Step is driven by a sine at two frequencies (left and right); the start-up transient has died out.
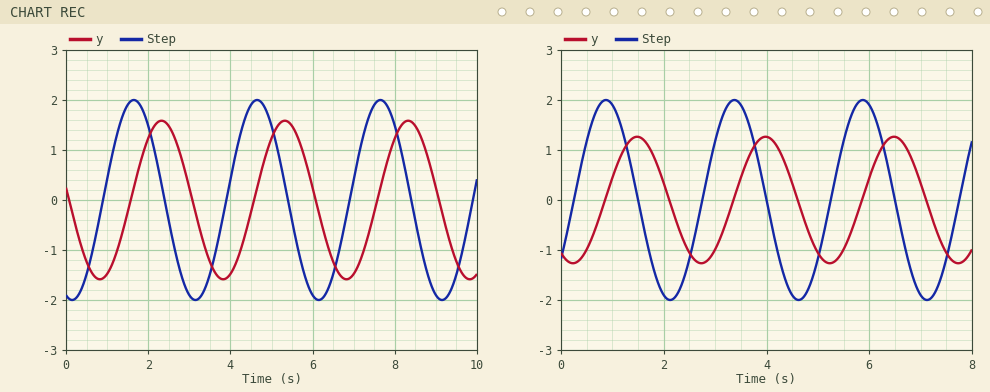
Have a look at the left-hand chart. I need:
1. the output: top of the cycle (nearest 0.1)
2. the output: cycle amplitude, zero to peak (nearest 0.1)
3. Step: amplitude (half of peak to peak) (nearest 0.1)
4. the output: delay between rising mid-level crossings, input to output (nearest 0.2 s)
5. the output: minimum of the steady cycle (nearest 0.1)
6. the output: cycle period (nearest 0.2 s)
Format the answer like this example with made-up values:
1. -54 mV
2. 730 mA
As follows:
1. 1.6
2. 1.6
3. 2.0
4. 0.6 s
5. -1.6
6. 3.0 s
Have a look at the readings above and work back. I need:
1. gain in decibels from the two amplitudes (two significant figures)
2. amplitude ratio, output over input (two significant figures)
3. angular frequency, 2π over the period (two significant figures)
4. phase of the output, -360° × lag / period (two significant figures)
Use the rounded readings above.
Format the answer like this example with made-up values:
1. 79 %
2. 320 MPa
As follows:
1. -1.9 dB
2. 0.80
3. 2.1 rad/s
4. -72°
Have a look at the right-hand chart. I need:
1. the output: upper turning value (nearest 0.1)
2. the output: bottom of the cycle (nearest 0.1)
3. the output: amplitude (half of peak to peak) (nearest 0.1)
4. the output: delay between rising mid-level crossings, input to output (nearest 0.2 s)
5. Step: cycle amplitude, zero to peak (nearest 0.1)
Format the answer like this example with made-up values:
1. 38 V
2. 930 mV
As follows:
1. 1.3
2. -1.3
3. 1.3
4. 0.6 s
5. 2.0
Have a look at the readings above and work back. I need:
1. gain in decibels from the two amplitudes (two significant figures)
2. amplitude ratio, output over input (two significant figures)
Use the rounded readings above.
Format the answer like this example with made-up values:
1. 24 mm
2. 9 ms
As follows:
1. -3.7 dB
2. 0.65
